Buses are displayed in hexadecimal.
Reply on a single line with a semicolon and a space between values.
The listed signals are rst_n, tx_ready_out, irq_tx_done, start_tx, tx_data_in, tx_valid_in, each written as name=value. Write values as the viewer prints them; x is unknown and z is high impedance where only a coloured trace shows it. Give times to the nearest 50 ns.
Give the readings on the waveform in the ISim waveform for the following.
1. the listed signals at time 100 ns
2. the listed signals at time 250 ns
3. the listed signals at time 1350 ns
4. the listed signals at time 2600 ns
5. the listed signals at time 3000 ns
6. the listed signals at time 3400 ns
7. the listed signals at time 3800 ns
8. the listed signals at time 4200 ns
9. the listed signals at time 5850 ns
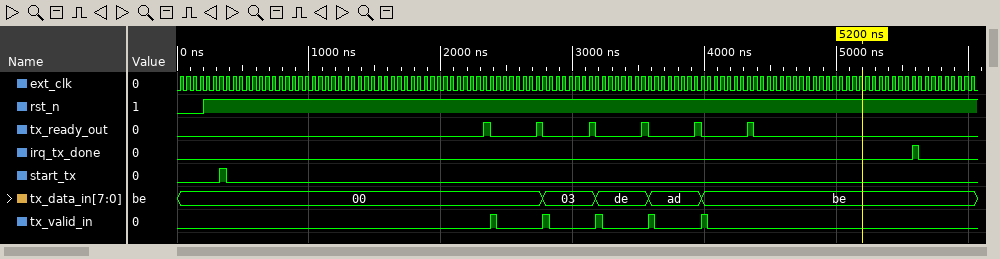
rst_n=0, tx_ready_out=0, irq_tx_done=0, start_tx=0, tx_data_in=00, tx_valid_in=0; rst_n=1, tx_ready_out=0, irq_tx_done=0, start_tx=0, tx_data_in=00, tx_valid_in=0; rst_n=1, tx_ready_out=0, irq_tx_done=0, start_tx=0, tx_data_in=00, tx_valid_in=0; rst_n=1, tx_ready_out=0, irq_tx_done=0, start_tx=0, tx_data_in=00, tx_valid_in=0; rst_n=1, tx_ready_out=0, irq_tx_done=0, start_tx=0, tx_data_in=03, tx_valid_in=0; rst_n=1, tx_ready_out=0, irq_tx_done=0, start_tx=0, tx_data_in=de, tx_valid_in=0; rst_n=1, tx_ready_out=0, irq_tx_done=0, start_tx=0, tx_data_in=ad, tx_valid_in=0; rst_n=1, tx_ready_out=0, irq_tx_done=0, start_tx=0, tx_data_in=be, tx_valid_in=0; rst_n=1, tx_ready_out=0, irq_tx_done=0, start_tx=0, tx_data_in=be, tx_valid_in=0
